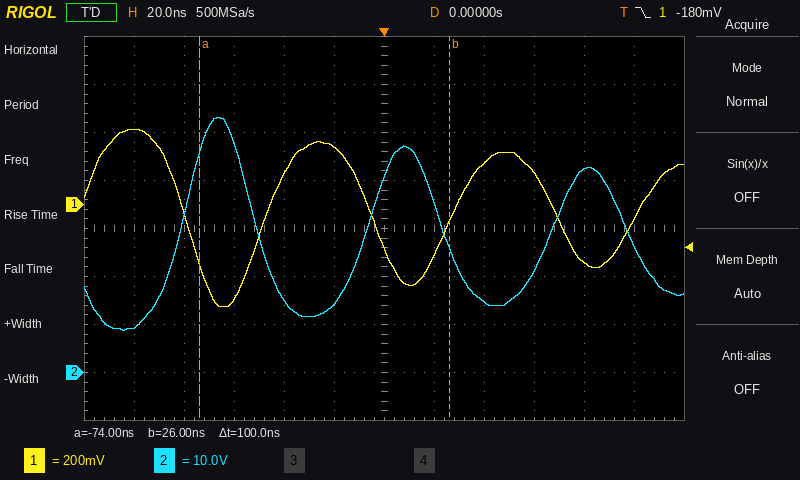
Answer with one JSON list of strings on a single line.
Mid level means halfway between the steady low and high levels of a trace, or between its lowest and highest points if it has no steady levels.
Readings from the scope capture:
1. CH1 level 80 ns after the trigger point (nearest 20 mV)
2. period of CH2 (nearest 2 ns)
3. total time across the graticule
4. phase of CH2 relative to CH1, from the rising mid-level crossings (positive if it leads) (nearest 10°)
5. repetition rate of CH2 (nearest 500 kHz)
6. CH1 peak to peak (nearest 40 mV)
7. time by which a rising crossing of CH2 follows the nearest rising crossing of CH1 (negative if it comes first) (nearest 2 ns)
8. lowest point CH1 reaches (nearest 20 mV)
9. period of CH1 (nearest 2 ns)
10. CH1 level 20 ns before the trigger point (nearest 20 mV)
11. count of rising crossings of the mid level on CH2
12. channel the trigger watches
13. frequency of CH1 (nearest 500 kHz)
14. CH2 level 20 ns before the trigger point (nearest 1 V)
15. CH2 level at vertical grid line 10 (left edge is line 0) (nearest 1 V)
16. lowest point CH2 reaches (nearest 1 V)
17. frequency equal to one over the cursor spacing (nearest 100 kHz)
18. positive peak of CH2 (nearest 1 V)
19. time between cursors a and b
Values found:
["-240 mV", "74 ns", "240 ns", "+160°", "13.5 MHz", "720 mV", "-32 ns", "-420 mV", "74 ns", "240 mV", "3", "CH1", "13.5 MHz", "14 V", "42 V", "9 V", "10.0 MHz", "53 V", "100 ns"]
